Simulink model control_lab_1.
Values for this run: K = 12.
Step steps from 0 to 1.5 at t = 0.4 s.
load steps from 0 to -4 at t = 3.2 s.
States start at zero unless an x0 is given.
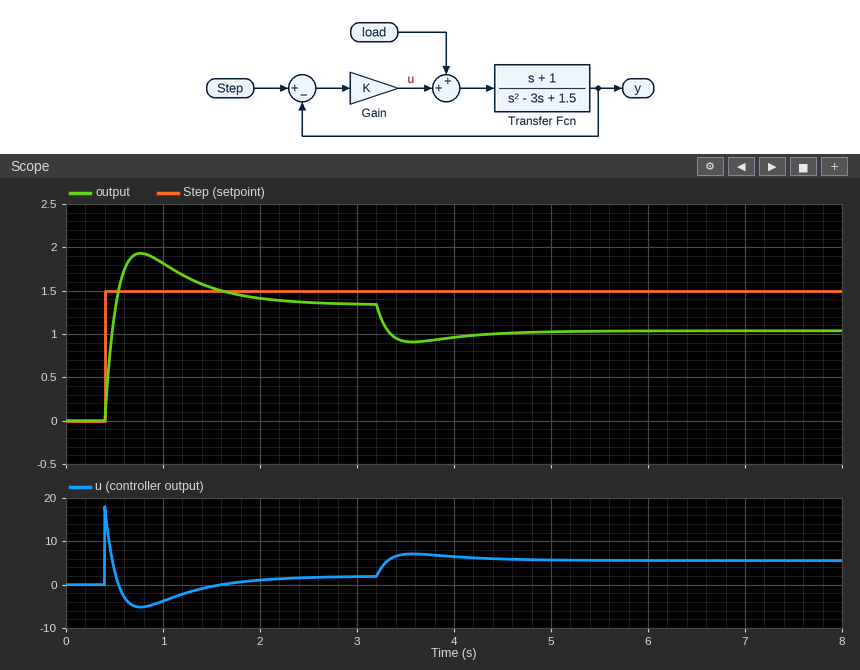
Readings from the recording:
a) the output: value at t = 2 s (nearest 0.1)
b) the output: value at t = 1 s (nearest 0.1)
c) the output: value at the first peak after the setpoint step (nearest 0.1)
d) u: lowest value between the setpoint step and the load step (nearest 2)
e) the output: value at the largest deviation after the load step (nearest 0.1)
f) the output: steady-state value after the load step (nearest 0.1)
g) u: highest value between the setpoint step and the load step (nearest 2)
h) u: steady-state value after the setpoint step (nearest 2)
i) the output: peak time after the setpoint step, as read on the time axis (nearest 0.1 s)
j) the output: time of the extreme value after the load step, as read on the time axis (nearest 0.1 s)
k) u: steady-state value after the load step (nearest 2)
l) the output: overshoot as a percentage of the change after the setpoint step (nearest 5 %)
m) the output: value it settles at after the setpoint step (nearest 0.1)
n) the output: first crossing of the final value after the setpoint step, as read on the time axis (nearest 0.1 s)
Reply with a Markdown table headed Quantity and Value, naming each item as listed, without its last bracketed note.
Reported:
| Quantity | Value |
|---|---|
| the output: value at t = 2 s | 1.4 |
| the output: value at t = 1 s | 1.8 |
| the output: value at the first peak after the setpoint step | 1.9 |
| u: lowest value between the setpoint step and the load step | -6 |
| the output: value at the largest deviation after the load step | 0.9 |
| the output: steady-state value after the load step | 1.0 |
| u: highest value between the setpoint step and the load step | 18 |
| u: steady-state value after the setpoint step | 2 |
| the output: peak time after the setpoint step, as read on the time axis | 0.8 s |
| the output: time of the extreme value after the load step, as read on the time axis | 3.6 s |
| u: steady-state value after the load step | 6 |
| the output: overshoot as a percentage of the change after the setpoint step | 45 % |
| the output: value it settles at after the setpoint step | 1.3 |
| the output: first crossing of the final value after the setpoint step, as read on the time axis | 0.5 s |
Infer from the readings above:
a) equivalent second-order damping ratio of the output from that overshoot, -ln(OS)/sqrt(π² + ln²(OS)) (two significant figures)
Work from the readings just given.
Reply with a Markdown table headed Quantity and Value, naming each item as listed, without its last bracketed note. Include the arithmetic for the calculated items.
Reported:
| Quantity | Value |
|---|---|
| equivalent second-order damping ratio of the output from that overshoot, -ln(OS)/sqrt(π² + ln²(OS)) | ln(0.45) = -0.799; 0.799 / sqrt(9.870 + 0.638) = 0.25 |
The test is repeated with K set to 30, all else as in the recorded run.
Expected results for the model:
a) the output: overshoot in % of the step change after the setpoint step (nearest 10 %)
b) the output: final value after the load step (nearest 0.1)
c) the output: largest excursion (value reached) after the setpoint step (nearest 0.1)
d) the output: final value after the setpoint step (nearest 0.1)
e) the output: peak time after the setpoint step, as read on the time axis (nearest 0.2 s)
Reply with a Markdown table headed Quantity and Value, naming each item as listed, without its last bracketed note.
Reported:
| Quantity | Value |
|---|---|
| the output: overshoot in % of the step change after the setpoint step | 20 % |
| the output: final value after the load step | 1.3 |
| the output: largest excursion (value reached) after the setpoint step | 1.7 |
| the output: final value after the setpoint step | 1.4 |
| the output: peak time after the setpoint step, as read on the time axis | 0.6 s |
